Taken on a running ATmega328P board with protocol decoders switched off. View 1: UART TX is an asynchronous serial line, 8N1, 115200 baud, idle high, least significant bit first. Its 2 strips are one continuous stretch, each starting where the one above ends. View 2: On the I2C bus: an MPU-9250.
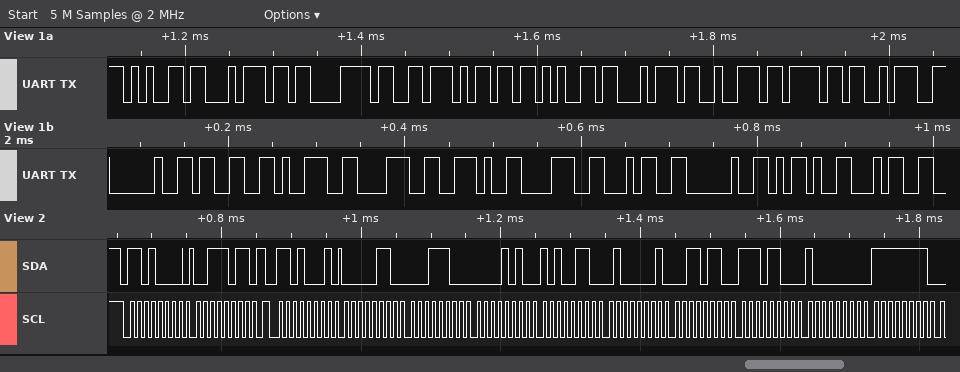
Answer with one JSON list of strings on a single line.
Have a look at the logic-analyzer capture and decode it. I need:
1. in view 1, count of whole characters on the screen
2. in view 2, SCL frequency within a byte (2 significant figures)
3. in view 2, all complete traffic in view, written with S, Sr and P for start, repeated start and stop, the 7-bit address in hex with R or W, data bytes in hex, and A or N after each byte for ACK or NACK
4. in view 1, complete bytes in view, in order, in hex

["20", "100 kHz", "S 68W A 3B A Sr 68R A 06 A 1C A 0A A A6 A 41 A 36 A EC A 80 A FF A", "65 74 C3 B3 6D 65 74 72 6F 3A 20 33 39 38 2E 38 34 20 2D 34"]
